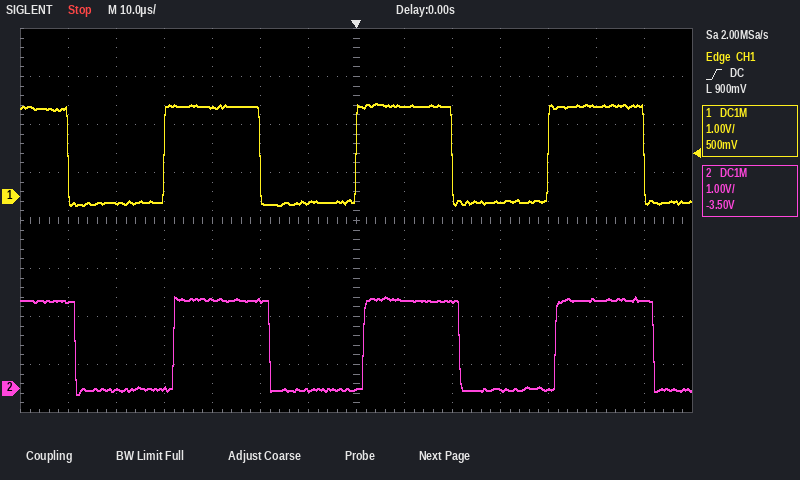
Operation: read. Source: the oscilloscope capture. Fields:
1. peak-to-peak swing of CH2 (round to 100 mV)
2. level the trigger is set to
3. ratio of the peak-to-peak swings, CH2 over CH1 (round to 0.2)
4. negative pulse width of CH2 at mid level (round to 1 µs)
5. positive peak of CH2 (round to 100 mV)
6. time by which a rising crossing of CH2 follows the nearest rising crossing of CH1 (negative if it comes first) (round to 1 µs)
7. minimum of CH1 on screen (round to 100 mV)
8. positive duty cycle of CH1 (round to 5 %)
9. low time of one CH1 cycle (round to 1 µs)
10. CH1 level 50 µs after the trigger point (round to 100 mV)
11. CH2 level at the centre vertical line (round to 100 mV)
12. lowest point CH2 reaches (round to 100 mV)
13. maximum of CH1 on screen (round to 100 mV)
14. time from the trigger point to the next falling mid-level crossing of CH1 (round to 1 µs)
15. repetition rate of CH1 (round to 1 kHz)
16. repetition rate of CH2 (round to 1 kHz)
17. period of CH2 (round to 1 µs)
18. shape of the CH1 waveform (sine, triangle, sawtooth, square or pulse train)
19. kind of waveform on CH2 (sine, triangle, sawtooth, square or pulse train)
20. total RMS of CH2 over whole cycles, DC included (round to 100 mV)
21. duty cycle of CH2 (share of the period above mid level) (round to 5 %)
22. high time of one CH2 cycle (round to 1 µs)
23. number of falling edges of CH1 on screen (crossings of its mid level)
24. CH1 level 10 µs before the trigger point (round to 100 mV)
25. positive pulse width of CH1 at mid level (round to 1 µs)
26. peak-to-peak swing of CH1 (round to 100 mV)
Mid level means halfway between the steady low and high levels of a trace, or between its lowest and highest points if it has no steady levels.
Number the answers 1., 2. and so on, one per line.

1. 2.0 V
2. 900 mV
3. 1.0
4. 20 µs
5. 1.9 V
6. +2 µs
7. -200 mV
8. 50 %
9. 20 µs
10. 1.9 V
11. 0.0 V
12. -100 mV
13. 1.9 V
14. 20 µs
15. 25 kHz
16. 25 kHz
17. 40 µs
18. square
19. square
20. 1.3 V
21. 50 %
22. 20 µs
23. 4
24. -100 mV
25. 20 µs
26. 2.1 V
